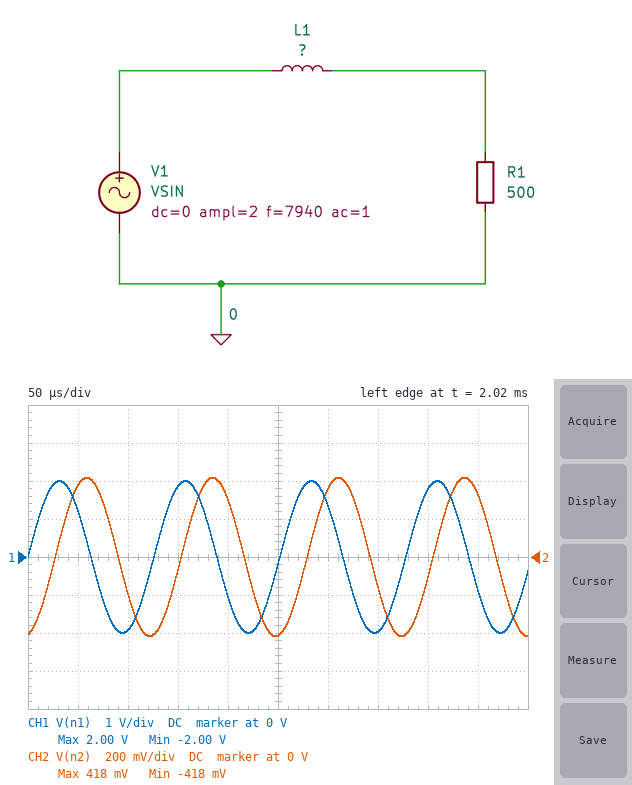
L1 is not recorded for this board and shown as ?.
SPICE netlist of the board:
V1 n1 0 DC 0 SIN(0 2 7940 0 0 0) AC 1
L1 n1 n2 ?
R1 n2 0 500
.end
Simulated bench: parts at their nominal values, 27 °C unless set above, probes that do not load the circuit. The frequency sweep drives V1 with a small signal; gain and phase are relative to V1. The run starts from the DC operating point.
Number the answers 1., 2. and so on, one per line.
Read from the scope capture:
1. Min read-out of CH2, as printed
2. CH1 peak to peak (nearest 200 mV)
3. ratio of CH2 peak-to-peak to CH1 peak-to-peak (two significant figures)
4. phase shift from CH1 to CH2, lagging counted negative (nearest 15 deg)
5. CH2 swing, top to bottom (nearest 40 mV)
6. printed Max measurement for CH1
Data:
1. -418 mV
2. 4.0 V
3. 0.21
4. -75 deg
5. 840 mV
6. 2.00 V
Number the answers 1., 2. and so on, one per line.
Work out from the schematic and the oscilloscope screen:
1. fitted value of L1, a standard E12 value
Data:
1. 47 mH
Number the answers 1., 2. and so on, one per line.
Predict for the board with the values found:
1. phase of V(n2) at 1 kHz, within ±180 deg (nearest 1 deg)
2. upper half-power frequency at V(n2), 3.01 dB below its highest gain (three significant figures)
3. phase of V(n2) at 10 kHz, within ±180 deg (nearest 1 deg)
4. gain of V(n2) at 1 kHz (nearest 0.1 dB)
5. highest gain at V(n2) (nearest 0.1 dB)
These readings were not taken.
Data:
1. -31 deg
2. 1.69 kHz
3. -80 deg
4. -1.3 dB
5. 0 dB
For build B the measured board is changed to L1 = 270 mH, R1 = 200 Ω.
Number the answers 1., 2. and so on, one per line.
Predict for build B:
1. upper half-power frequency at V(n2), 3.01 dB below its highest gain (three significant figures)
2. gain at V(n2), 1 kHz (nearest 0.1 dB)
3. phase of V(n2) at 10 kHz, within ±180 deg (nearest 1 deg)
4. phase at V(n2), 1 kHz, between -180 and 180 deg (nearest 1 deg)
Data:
1. 118 Hz
2. -18.6 dB
3. -89 deg
4. -83 deg
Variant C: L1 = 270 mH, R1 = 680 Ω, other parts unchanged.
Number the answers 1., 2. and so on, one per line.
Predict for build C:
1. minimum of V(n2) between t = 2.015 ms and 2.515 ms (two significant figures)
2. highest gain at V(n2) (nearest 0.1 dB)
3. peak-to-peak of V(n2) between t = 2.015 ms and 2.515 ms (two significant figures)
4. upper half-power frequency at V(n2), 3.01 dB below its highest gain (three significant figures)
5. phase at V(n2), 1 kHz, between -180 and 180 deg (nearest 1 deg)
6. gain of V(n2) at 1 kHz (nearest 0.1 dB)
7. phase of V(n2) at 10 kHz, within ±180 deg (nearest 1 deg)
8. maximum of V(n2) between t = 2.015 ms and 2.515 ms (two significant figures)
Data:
1. -100 mV
2. 0 dB
3. 200 mV
4. 401 Hz
5. -68 deg
6. -8.6 dB
7. -88 deg
8. 100 mV
